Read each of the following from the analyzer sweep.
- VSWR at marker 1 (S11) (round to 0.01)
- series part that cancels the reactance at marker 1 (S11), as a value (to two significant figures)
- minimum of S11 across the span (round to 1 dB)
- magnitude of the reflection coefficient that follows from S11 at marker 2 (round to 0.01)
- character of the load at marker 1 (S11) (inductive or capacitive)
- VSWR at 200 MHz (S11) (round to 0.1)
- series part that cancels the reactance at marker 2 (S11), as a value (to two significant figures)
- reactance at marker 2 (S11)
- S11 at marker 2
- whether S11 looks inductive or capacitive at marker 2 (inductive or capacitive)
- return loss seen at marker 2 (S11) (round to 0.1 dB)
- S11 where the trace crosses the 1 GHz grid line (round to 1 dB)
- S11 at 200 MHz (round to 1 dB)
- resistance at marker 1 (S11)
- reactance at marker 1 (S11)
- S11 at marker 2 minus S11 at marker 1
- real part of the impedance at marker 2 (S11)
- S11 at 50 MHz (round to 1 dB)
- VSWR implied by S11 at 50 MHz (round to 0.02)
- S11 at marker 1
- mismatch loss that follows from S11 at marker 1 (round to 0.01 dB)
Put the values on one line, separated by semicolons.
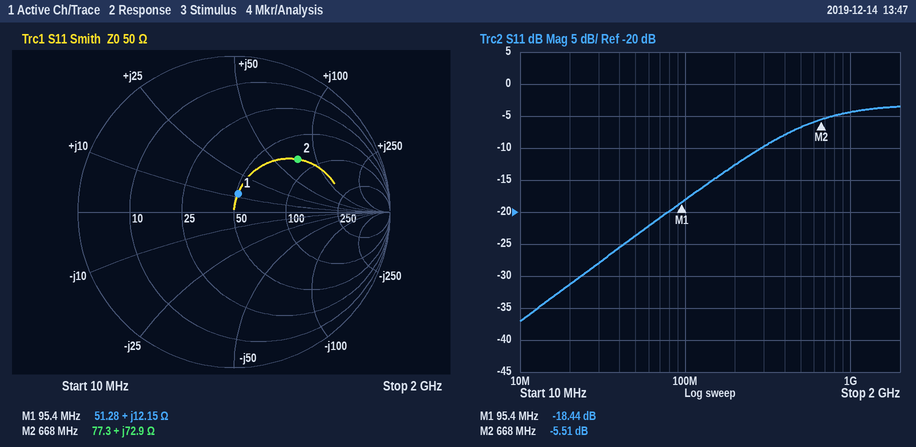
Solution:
1.27; 140 pF; -37 dB; 0.53; inductive; 1.6; 3.3 pF; +72.9 Ω; -5.51 dB; inductive; 5.5 dB; -4 dB; -13 dB; 51.28 Ω; +12.15 Ω; 12.93 dB; 77.3 Ω; -24 dB; 1.14; -18.44 dB; 0.06 dB
